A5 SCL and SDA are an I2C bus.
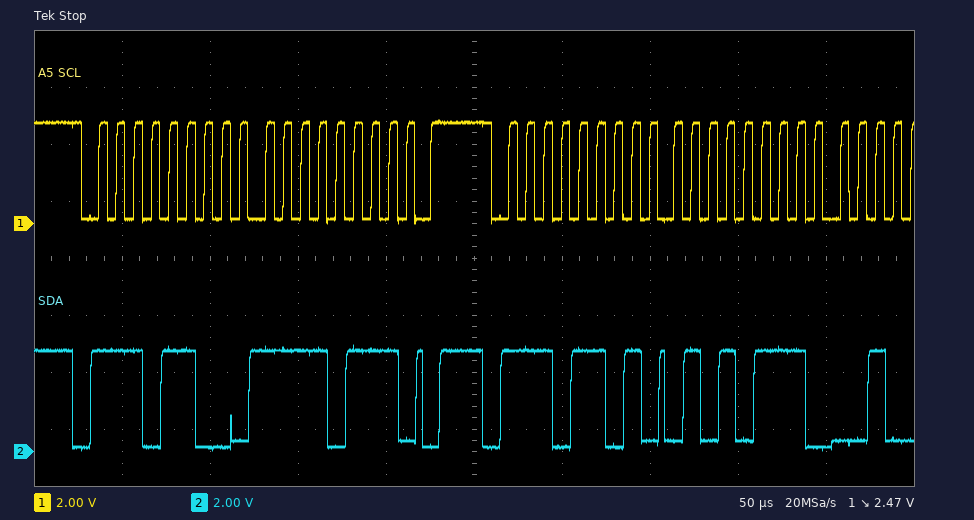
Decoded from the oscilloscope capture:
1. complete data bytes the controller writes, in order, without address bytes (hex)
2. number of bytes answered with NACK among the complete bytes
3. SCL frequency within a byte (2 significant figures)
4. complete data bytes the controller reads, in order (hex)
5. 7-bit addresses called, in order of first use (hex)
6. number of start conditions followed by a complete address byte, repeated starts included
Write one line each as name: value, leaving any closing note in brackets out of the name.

complete data bytes the controller writes, in order, without address bytes: F7
number of bytes answered with NACK among the complete bytes: 0
SCL frequency within a byte: 100 kHz
complete data bytes the controller reads, in order: 57
7-bit addresses called, in order of first use: 0x76
number of start conditions followed by a complete address byte, repeated starts included: 2
